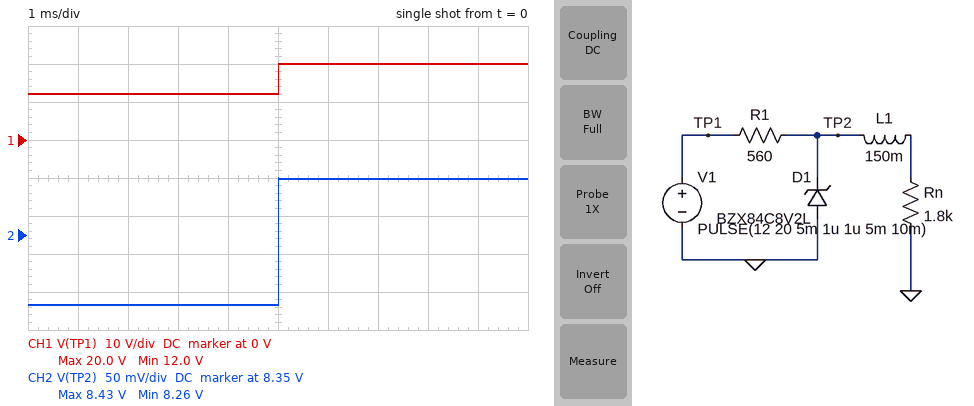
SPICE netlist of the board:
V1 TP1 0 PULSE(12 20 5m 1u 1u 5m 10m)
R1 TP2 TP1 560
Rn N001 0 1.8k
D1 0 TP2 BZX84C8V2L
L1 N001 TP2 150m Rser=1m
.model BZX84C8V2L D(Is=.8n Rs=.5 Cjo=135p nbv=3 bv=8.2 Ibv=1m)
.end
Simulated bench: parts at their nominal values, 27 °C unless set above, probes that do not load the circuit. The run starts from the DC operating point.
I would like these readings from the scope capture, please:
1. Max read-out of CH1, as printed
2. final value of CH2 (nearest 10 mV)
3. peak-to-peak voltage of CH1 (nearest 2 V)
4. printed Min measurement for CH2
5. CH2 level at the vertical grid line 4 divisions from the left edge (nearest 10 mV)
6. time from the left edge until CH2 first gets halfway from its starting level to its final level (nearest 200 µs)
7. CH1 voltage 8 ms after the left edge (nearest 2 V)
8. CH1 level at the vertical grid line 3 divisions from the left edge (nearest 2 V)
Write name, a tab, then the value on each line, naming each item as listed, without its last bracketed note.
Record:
Max read-out of CH1, as printed	20.0 V
final value of CH2	8.42 V
peak-to-peak voltage of CH1	8 V
printed Min measurement for CH2	8.26 V
CH2 level at the vertical grid line 4 divisions from the left edge	8.26 V
time from the left edge until CH2 first gets halfway from its starting level to its final level	5.0 ms
CH1 voltage 8 ms after the left edge	20 V
CH1 level at the vertical grid line 3 divisions from the left edge	12 V
